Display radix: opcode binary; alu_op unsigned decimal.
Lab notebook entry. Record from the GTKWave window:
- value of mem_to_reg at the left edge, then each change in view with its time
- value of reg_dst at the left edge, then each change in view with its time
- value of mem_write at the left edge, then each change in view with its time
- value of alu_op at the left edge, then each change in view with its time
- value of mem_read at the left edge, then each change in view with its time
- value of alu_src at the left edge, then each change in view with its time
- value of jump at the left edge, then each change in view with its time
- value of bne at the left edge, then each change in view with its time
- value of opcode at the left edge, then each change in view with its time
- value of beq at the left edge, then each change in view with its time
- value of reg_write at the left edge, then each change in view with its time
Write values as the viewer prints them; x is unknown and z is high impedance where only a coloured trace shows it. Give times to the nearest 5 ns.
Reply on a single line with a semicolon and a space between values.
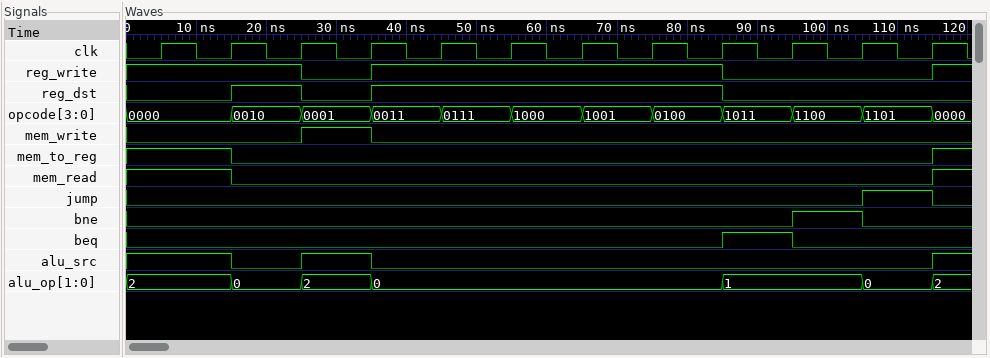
1, 0 at 15 ns, 1 at 115 ns; 0, 1 at 15 ns, 0 at 25 ns, 1 at 35 ns, 0 at 85 ns; 0, 1 at 25 ns, 0 at 35 ns; 2, 0 at 15 ns, 2 at 25 ns, 0 at 35 ns, 1 at 85 ns, 0 at 105 ns, 2 at 115 ns; 1, 0 at 15 ns, 1 at 115 ns; 1, 0 at 15 ns, 1 at 25 ns, 0 at 35 ns, 1 at 115 ns; 0, 1 at 105 ns, 0 at 115 ns; 0, 1 at 95 ns, 0 at 105 ns; 0000, 0010 at 15 ns, 0001 at 25 ns, 0011 at 35 ns, 0111 at 45 ns, 1000 at 55 ns, 1001 at 65 ns, 0100 at 75 ns, 1011 at 85 ns, 1100 at 95 ns, 1101 at 105 ns, 0000 at 115 ns; 0, 1 at 85 ns, 0 at 95 ns; 1, 0 at 25 ns, 1 at 35 ns, 0 at 85 ns, 1 at 115 ns
